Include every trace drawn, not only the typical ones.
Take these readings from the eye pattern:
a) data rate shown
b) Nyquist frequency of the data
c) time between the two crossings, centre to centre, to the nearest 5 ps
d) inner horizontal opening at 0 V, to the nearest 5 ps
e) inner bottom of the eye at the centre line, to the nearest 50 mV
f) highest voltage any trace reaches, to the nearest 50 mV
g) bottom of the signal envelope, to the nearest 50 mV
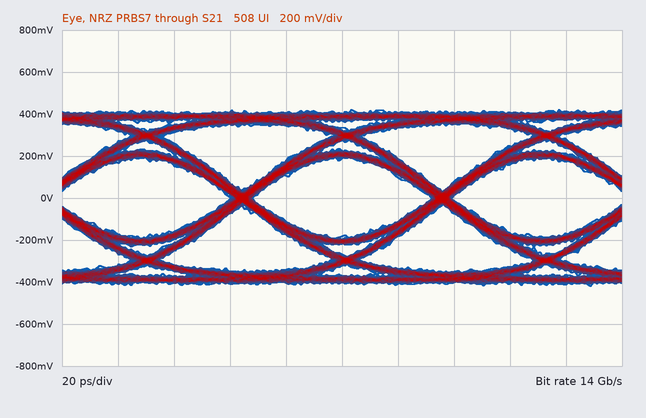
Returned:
14 Gb/s
7 GHz
70 ps
65 ps
-200 mV
400 mV
-400 mV
